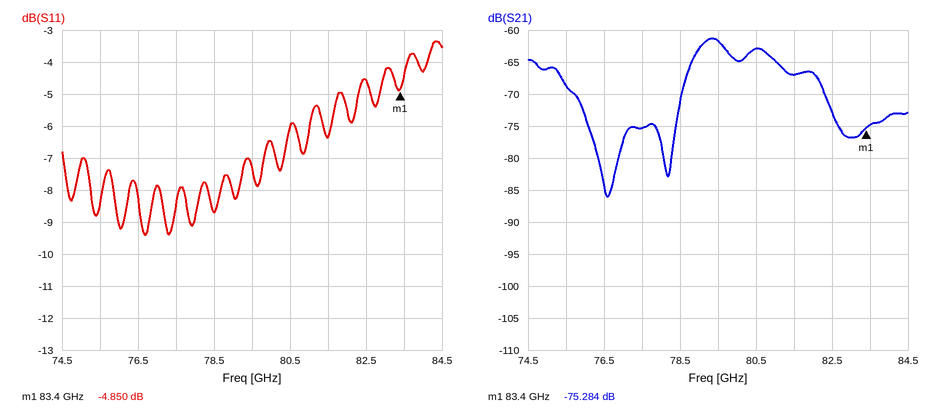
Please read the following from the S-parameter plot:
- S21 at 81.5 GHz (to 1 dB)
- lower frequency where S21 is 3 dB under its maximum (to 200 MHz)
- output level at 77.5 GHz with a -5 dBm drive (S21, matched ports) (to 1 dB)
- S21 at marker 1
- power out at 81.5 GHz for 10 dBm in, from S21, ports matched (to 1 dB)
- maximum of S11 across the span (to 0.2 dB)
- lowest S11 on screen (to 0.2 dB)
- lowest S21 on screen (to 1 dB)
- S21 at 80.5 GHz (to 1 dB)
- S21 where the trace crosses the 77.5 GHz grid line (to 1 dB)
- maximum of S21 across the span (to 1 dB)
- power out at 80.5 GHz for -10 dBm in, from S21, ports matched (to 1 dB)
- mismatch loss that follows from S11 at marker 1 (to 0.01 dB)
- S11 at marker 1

-67 dB
78.8 GHz
-80 dBm
-75.284 dB
-57 dBm
-3.4 dB
-9.4 dB
-86 dB
-63 dB
-75 dB
-61 dB
-73 dBm
1.72 dB
-4.850 dB
